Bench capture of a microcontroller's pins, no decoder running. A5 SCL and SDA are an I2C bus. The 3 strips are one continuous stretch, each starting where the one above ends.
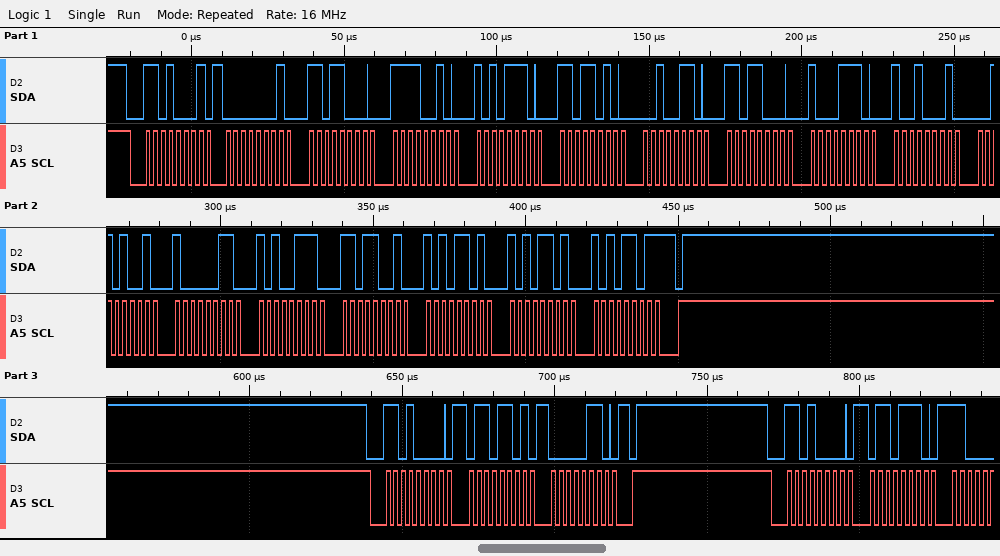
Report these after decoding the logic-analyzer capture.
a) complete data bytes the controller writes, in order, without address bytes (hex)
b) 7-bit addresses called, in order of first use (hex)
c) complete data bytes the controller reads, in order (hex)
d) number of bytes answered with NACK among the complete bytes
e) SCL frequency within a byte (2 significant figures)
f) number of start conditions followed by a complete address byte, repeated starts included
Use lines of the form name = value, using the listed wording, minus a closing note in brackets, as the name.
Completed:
complete data bytes the controller writes, in order, without address bytes = 6D 06 6E
7-bit addresses called, in order of first use = 0x68
complete data bytes the controller reads, in order = 01 D8 F2 AE DA 26 D8 8E 91 29 83 A7 D9 AD AD AD
number of bytes answered with NACK among the complete bytes = 1
SCL frequency within a byte = 400 kHz
number of start conditions followed by a complete address byte, repeated starts included = 3
